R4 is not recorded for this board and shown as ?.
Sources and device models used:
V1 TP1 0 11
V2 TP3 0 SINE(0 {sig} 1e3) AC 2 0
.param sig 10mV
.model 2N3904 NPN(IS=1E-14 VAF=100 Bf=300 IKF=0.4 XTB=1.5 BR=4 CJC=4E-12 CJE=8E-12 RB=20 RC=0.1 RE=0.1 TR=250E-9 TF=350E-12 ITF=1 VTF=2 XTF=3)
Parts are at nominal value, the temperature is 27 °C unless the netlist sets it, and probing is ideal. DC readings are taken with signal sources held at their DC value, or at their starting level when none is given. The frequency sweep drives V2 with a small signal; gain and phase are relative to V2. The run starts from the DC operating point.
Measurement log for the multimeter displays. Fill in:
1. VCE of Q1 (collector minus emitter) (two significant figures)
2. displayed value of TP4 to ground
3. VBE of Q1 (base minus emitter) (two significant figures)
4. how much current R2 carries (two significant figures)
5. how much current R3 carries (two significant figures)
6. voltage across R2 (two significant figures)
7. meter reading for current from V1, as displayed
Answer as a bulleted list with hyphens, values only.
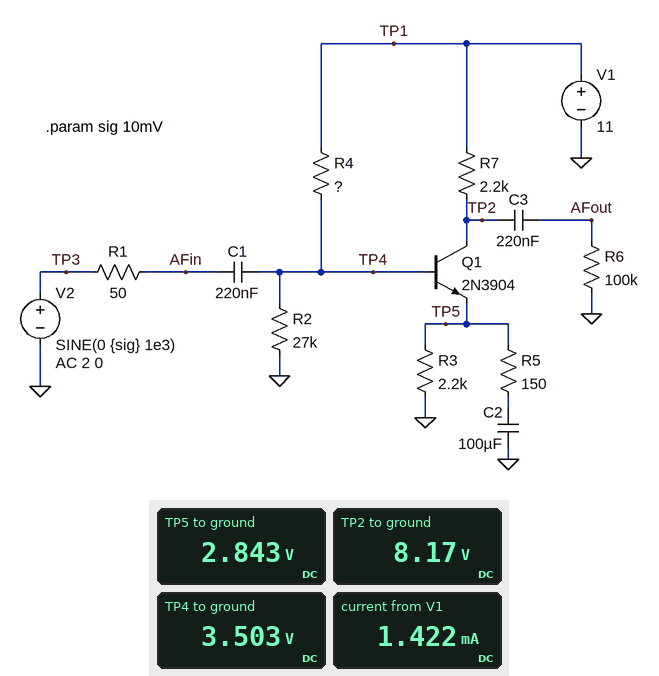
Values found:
- 5.3 V
- 3.503 V
- 660 mV
- 130 µA
- 1.3 mA
- 3.5 V
- 1.422 mA
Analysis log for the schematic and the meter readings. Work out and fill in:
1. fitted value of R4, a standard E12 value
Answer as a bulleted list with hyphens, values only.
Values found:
- 56 kΩ
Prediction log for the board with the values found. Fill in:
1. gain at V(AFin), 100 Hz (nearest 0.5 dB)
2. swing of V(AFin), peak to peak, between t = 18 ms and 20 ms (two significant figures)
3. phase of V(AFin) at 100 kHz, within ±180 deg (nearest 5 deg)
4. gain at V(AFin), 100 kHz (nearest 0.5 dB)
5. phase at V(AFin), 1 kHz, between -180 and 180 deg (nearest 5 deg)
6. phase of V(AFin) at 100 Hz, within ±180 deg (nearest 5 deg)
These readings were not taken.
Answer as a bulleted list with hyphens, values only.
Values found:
- 0 dB
- 20 mV
- 0 deg
- 0 dB
- 0 deg
- 0 deg
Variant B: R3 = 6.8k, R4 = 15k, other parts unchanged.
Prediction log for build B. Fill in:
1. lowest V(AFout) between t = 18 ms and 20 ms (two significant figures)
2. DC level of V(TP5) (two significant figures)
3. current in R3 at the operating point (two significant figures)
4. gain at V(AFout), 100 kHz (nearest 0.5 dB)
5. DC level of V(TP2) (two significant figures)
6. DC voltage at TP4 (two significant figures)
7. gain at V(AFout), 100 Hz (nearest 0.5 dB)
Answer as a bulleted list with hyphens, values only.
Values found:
- -120 mV
- 6.4 V
- 940 µA
- 21.5 dB
- 8.9 V
- 7.0 V
- 19.0 dB
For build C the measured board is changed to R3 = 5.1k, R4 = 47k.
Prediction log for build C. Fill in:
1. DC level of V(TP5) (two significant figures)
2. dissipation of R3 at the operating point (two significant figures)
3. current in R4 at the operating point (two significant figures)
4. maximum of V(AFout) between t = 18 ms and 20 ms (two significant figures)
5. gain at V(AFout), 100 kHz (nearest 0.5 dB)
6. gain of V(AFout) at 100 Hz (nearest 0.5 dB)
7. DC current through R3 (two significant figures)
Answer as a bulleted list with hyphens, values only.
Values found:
- 3.3 V
- 2.2 mW
- 150 µA
- 110 mV
- 21.0 dB
- 20.0 dB
- 650 µA
